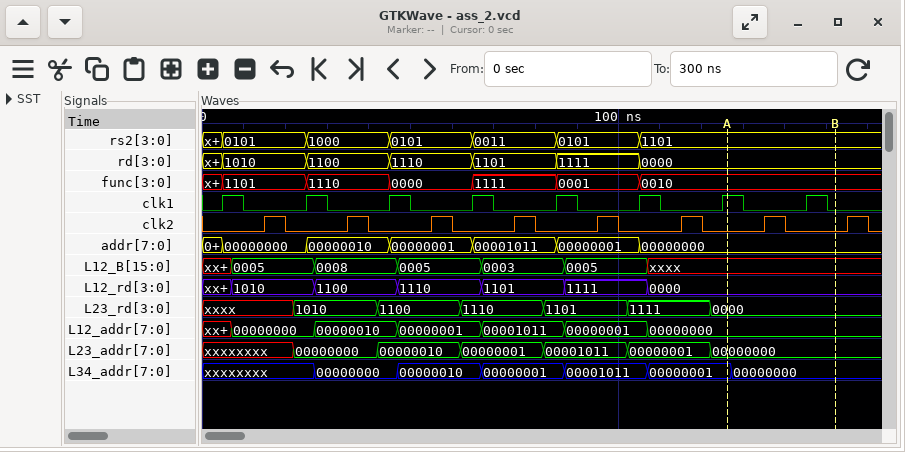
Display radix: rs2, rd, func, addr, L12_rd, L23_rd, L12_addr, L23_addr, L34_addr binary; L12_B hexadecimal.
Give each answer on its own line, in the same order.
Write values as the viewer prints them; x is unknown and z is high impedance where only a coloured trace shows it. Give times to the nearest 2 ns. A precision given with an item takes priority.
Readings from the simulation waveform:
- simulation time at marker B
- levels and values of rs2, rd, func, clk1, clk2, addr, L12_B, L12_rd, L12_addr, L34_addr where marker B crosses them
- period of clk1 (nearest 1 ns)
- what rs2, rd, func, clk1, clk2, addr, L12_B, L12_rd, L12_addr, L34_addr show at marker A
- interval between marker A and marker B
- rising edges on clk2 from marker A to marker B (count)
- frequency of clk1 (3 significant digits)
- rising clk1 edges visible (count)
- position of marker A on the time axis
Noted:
152 ns
rs2=1101, rd=0000, func=0010, clk1=0, clk2=0, addr=00000000, L12_B=xxxx, L12_rd=0000, L12_addr=00000000, L34_addr=00000000
20 ns
rs2=1101, rd=0000, func=0010, clk1=1, clk2=0, addr=00000000, L12_B=xxxx, L12_rd=0000, L12_addr=00000000, L34_addr=00000001
26 ns
1
50.0 MHz
8
126 ns
